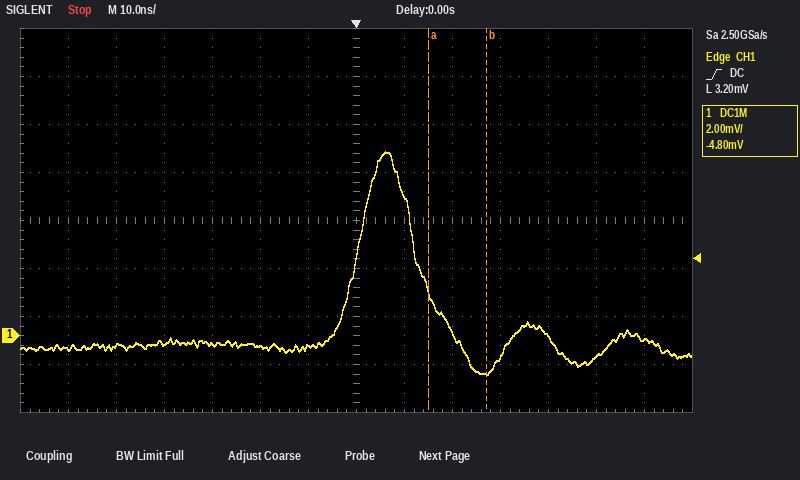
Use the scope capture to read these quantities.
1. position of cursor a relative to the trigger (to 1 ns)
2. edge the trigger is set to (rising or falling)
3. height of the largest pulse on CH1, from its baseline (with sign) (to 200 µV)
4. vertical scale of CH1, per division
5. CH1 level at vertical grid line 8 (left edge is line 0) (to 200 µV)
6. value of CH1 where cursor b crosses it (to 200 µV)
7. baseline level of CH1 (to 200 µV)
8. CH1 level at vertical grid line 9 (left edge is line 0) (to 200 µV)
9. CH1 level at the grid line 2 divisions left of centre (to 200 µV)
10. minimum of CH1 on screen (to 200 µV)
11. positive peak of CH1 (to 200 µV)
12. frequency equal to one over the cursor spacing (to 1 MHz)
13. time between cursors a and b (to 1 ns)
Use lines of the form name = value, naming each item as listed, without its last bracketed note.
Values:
position of cursor a relative to the trigger = +15 ns
edge the trigger is set to = rising
height of the largest pulse on CH1, from its baseline (with sign) = +8.0 mV
vertical scale of CH1, per division = 2 mV
CH1 level at vertical grid line 8 (left edge is line 0) = 5.8 mV
value of CH1 where cursor b crosses it = -1.6 mV
baseline level of CH1 = -400 µV
CH1 level at vertical grid line 9 (left edge is line 0) = 200 µV
CH1 level at the grid line 2 divisions left of centre = -400 µV
minimum of CH1 on screen = -1.6 mV
positive peak of CH1 = 7.6 mV
frequency equal to one over the cursor spacing = 83 MHz
time between cursors a and b = 12 ns
